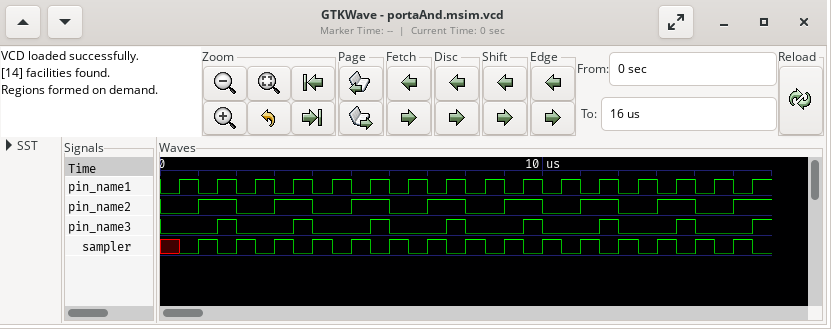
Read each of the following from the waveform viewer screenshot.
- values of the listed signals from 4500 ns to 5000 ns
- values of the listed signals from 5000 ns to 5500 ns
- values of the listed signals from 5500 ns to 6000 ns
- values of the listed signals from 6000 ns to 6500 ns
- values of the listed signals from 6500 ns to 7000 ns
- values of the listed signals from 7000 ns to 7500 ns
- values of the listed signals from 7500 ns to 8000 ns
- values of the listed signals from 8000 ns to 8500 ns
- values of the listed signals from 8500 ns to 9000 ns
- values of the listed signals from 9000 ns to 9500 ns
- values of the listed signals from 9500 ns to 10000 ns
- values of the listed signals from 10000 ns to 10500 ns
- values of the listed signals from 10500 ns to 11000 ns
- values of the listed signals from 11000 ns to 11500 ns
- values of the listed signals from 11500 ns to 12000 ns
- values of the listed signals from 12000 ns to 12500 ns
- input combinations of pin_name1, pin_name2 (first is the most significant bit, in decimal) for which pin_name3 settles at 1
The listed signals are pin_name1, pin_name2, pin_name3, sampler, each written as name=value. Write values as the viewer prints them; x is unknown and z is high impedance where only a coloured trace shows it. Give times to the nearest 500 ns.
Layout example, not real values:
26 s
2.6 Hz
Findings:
pin_name1=1, pin_name2=0, pin_name3=0, sampler=0
pin_name1=0, pin_name2=1, pin_name3=0, sampler=1
pin_name1=1, pin_name2=1, pin_name3=1, sampler=0
pin_name1=0, pin_name2=0, pin_name3=0, sampler=1
pin_name1=1, pin_name2=0, pin_name3=0, sampler=0
pin_name1=0, pin_name2=1, pin_name3=0, sampler=1
pin_name1=1, pin_name2=1, pin_name3=1, sampler=0
pin_name1=0, pin_name2=0, pin_name3=0, sampler=1
pin_name1=1, pin_name2=0, pin_name3=0, sampler=0
pin_name1=0, pin_name2=1, pin_name3=0, sampler=1
pin_name1=1, pin_name2=1, pin_name3=1, sampler=0
pin_name1=0, pin_name2=0, pin_name3=0, sampler=1
pin_name1=1, pin_name2=0, pin_name3=0, sampler=0
pin_name1=0, pin_name2=1, pin_name3=0, sampler=1
pin_name1=1, pin_name2=1, pin_name3=1, sampler=0
pin_name1=0, pin_name2=0, pin_name3=0, sampler=1
3
